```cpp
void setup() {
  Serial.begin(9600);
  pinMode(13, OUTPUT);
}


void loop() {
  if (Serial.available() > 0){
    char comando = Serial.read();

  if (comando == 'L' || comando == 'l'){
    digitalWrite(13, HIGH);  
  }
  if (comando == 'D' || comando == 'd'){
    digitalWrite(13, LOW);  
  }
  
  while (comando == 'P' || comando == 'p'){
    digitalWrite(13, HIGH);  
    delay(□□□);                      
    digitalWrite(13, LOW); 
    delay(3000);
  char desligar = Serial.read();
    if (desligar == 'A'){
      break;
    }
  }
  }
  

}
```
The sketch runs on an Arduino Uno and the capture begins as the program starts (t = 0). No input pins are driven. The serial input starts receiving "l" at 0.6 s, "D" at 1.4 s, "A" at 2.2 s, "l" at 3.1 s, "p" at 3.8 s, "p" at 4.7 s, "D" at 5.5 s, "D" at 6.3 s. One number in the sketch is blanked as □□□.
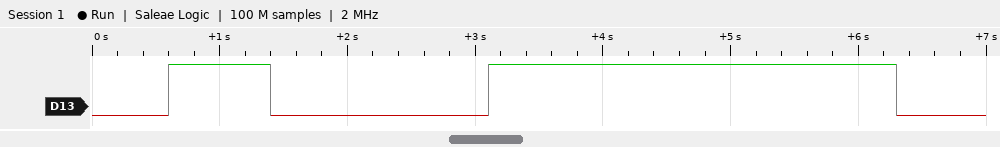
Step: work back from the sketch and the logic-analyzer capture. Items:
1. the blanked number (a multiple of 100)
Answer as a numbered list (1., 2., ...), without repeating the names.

1. 2500
